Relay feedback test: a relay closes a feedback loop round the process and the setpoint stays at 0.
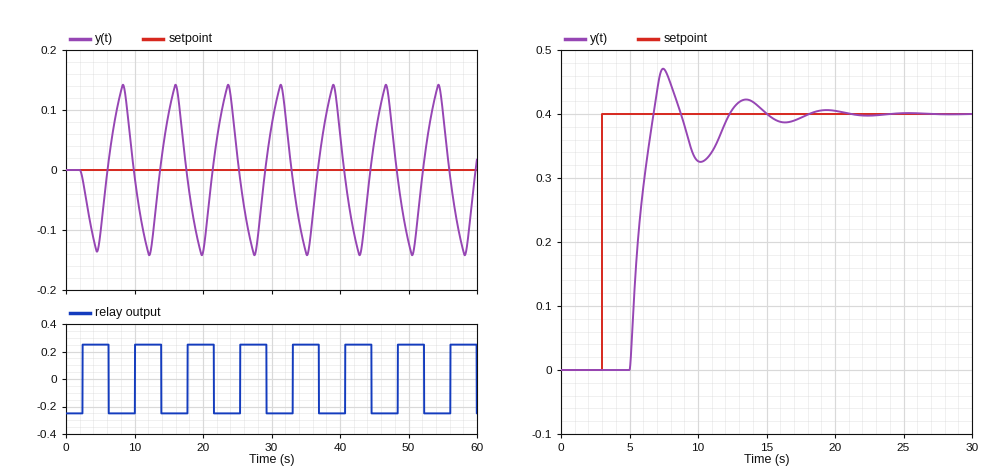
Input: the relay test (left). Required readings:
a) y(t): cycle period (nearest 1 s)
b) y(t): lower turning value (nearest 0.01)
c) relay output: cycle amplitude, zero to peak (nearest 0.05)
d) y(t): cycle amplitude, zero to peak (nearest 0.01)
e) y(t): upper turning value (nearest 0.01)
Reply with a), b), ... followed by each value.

a) 8 s
b) -0.14
c) 0.25
d) 0.14
e) 0.14
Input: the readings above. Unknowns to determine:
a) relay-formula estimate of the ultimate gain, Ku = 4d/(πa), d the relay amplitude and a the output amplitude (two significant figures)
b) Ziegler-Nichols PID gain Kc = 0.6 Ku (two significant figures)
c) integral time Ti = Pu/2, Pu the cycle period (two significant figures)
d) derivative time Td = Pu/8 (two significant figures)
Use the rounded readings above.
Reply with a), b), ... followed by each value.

a) 2.3
b) 1.4
c) 4.0 s
d) 1.0 s
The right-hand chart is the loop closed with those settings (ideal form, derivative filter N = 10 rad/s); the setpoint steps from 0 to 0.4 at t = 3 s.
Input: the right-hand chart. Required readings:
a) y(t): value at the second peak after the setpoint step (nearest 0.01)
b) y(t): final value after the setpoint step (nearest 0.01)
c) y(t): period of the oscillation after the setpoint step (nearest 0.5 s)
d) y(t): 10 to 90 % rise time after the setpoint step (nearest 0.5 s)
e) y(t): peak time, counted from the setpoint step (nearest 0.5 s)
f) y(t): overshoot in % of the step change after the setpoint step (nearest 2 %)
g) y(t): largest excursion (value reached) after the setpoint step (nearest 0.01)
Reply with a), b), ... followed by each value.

a) 0.42
b) 0.40
c) 6.0 s
d) 1.5 s
e) 4.5 s
f) 18 %
g) 0.47
